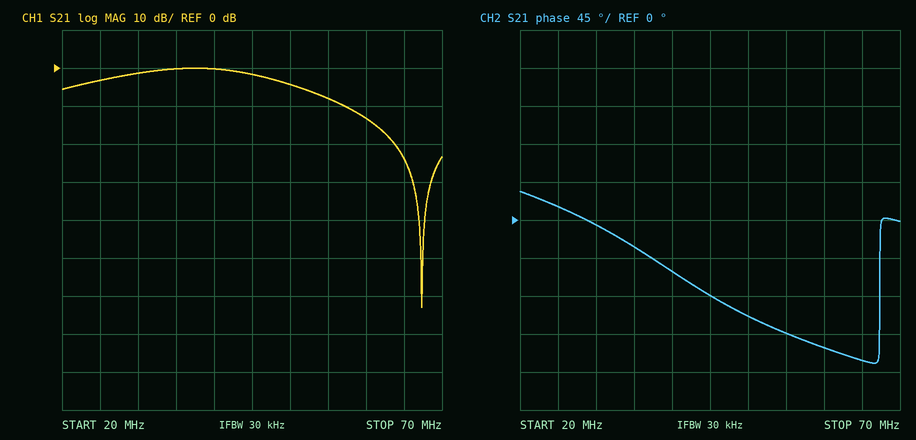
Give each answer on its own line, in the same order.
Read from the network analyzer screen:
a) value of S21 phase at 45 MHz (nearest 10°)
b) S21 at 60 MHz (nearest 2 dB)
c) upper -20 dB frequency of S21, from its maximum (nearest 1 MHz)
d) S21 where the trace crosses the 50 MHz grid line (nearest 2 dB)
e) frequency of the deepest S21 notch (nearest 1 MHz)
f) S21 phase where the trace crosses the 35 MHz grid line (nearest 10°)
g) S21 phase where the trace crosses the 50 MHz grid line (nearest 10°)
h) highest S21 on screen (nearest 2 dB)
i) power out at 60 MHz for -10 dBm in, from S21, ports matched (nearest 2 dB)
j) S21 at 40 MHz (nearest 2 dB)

-90°
-14 dB
64 MHz
-4 dB
67 MHz
-30°
-110°
0 dB
-24 dBm
0 dB
